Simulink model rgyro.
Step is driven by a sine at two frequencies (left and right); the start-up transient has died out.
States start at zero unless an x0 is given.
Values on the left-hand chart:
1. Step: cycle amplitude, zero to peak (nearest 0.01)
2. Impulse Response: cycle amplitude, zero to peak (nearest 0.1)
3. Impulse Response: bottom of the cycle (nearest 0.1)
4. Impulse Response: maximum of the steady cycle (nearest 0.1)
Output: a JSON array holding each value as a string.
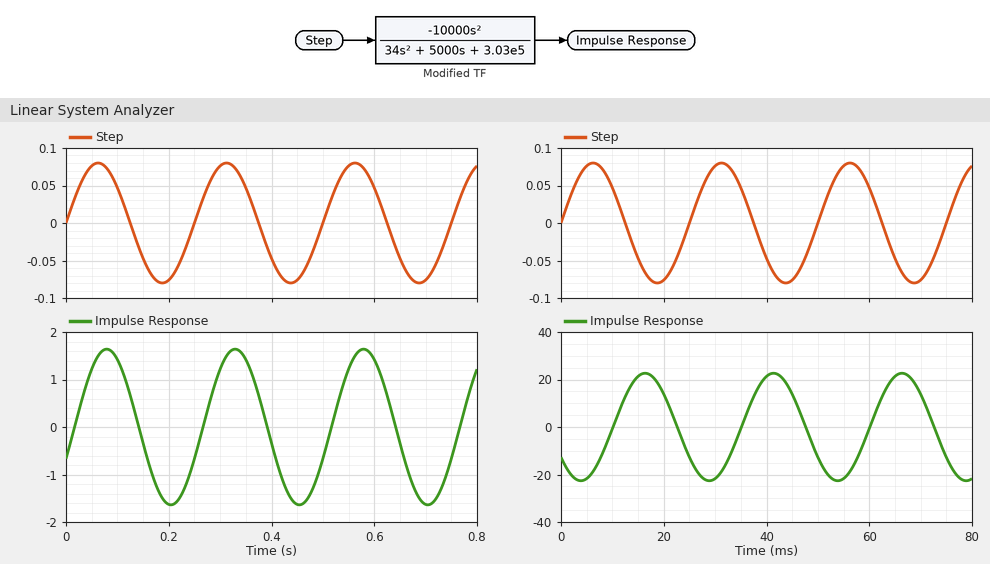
["0.08", "1.6", "-1.6", "1.6"]
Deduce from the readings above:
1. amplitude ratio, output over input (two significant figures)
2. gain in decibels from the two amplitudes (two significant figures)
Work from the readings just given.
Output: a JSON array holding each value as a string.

["20", "26 dB"]
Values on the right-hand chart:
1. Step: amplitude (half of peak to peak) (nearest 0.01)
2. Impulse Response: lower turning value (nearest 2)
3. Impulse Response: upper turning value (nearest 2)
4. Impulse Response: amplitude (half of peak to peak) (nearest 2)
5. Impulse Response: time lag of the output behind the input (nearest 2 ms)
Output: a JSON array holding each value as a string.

["0.08", "-22", "22", "22", "10 ms"]
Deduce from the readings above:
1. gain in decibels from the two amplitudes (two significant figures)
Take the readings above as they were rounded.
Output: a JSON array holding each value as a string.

["49 dB"]
